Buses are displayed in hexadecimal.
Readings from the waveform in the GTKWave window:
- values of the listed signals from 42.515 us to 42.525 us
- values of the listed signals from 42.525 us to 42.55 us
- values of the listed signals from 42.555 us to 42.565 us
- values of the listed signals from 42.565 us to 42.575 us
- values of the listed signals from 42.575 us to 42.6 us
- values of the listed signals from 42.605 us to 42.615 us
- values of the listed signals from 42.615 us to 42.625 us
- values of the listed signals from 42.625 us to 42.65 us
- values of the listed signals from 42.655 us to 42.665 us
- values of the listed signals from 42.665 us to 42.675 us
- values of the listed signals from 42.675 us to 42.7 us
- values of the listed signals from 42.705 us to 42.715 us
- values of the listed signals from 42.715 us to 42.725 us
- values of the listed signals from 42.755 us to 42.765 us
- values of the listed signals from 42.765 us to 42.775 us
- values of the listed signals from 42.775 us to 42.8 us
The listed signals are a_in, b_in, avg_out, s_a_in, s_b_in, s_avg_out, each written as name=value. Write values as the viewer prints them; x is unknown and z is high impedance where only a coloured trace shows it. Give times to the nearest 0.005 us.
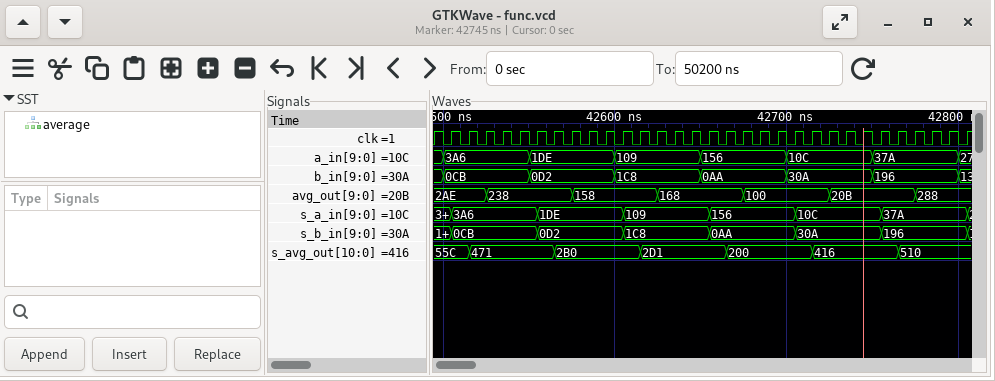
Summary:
a_in=3A6, b_in=0CB, avg_out=2AE, s_a_in=3A6, s_b_in=0CB, s_avg_out=471
a_in=3A6, b_in=0CB, avg_out=238, s_a_in=3A6, s_b_in=0CB, s_avg_out=471
a_in=1DE, b_in=0D2, avg_out=238, s_a_in=1DE, s_b_in=0D2, s_avg_out=471
a_in=1DE, b_in=0D2, avg_out=238, s_a_in=1DE, s_b_in=0D2, s_avg_out=2B0
a_in=1DE, b_in=0D2, avg_out=158, s_a_in=1DE, s_b_in=0D2, s_avg_out=2B0
a_in=109, b_in=1C8, avg_out=158, s_a_in=109, s_b_in=1C8, s_avg_out=2B0
a_in=109, b_in=1C8, avg_out=158, s_a_in=109, s_b_in=1C8, s_avg_out=2D1
a_in=109, b_in=1C8, avg_out=168, s_a_in=109, s_b_in=1C8, s_avg_out=2D1
a_in=156, b_in=0AA, avg_out=168, s_a_in=156, s_b_in=0AA, s_avg_out=2D1
a_in=156, b_in=0AA, avg_out=168, s_a_in=156, s_b_in=0AA, s_avg_out=200
a_in=156, b_in=0AA, avg_out=100, s_a_in=156, s_b_in=0AA, s_avg_out=200
a_in=10C, b_in=30A, avg_out=100, s_a_in=10C, s_b_in=30A, s_avg_out=200
a_in=10C, b_in=30A, avg_out=100, s_a_in=10C, s_b_in=30A, s_avg_out=416
a_in=37A, b_in=196, avg_out=20B, s_a_in=37A, s_b_in=196, s_avg_out=416
a_in=37A, b_in=196, avg_out=20B, s_a_in=37A, s_b_in=196, s_avg_out=510
a_in=37A, b_in=196, avg_out=288, s_a_in=37A, s_b_in=196, s_avg_out=510
